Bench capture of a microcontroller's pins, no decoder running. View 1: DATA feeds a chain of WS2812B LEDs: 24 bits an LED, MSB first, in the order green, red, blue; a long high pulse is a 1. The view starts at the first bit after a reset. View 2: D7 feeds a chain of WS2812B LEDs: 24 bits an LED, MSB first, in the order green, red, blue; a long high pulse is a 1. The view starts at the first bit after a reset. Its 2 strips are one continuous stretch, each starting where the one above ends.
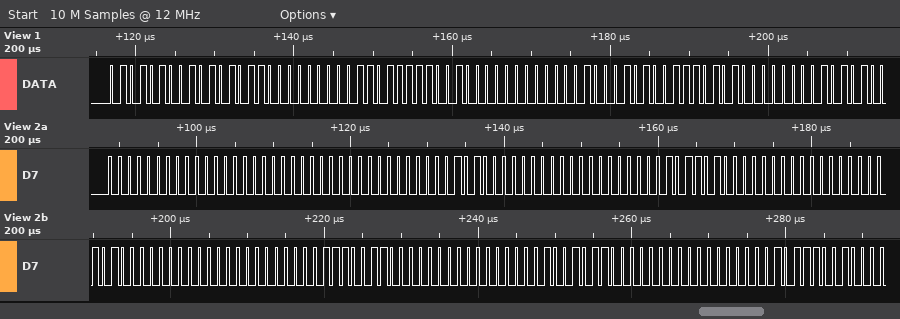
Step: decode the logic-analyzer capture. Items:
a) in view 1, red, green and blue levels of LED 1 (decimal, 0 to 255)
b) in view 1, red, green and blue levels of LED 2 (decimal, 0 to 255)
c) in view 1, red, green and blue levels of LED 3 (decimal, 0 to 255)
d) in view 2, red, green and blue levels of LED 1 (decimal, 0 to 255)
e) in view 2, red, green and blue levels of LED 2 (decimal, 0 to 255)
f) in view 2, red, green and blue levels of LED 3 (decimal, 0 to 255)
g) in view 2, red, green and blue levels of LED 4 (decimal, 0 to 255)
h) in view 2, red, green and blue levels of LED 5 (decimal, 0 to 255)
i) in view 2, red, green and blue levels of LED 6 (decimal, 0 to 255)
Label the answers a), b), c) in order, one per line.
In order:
a) 171, 84, 0
b) 144, 111, 0
c) 117, 138, 0
d) 0, 0, 0
e) 10, 0, 0
f) 45, 0, 0
g) 80, 0, 0
h) 115, 0, 0
i) 150, 0, 0
